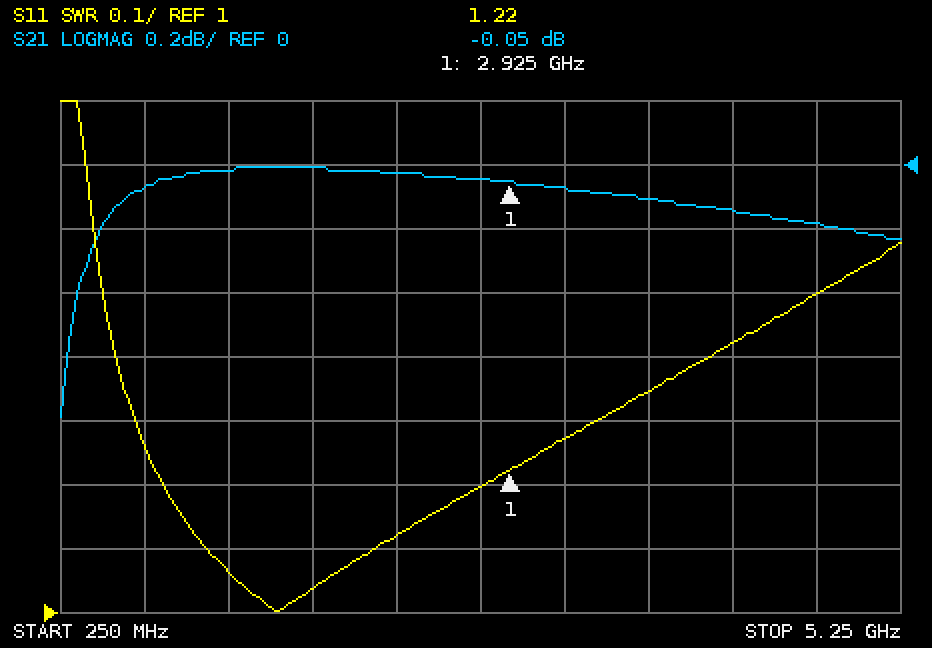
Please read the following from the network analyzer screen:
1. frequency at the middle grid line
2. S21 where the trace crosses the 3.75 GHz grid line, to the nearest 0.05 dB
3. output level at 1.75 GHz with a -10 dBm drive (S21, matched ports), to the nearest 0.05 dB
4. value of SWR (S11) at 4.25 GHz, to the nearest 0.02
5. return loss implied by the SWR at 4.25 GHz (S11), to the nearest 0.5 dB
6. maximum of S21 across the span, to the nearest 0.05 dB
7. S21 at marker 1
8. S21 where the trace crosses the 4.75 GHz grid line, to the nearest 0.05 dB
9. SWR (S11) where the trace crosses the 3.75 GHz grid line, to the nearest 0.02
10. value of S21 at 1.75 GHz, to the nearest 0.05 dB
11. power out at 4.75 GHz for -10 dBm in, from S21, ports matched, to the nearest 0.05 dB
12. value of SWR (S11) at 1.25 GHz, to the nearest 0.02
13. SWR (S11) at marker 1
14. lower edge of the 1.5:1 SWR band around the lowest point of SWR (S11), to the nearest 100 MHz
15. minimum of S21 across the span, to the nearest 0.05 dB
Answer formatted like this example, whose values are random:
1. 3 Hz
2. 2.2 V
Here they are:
1. 2.75 GHz
2. -0.10 dB
3. -10.00 dBm
4. 1.42
5. 15.0 dB
6. 0.00 dB
7. -0.05 dB
8. -0.20 dB
9. 1.34
10. 0.00 dB
11. -10.20 dBm
12. 1.06
13. 1.22
14. 500 MHz
15. -0.80 dB
